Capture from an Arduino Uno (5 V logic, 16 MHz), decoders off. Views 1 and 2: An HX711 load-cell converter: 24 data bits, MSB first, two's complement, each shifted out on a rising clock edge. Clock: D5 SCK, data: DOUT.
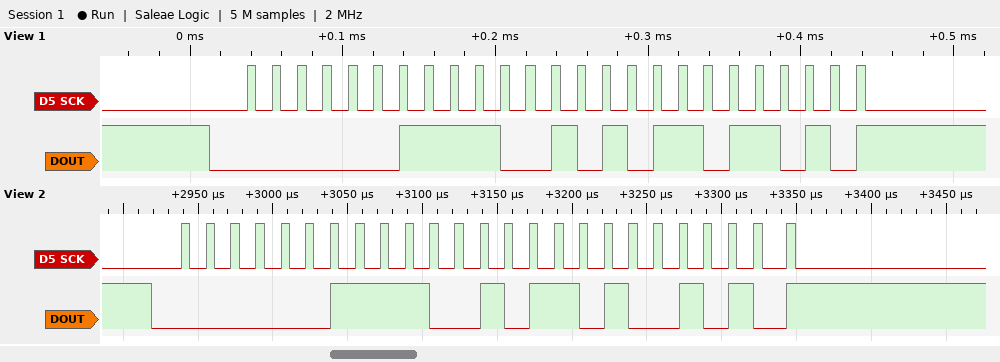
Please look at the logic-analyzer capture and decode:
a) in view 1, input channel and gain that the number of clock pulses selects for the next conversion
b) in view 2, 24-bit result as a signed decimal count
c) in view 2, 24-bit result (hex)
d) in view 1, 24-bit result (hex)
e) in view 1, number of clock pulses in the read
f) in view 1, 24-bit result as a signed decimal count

channel A, gain 128
248650
0x03CB4A
0x03CADA
25
248538
